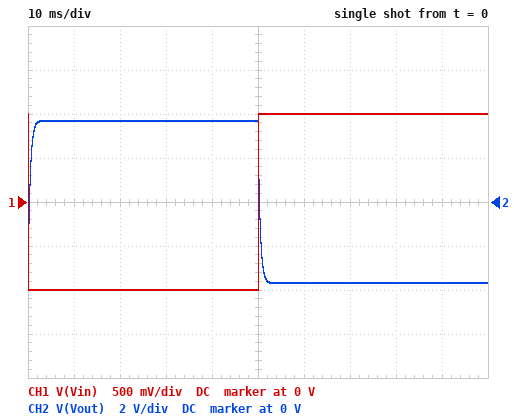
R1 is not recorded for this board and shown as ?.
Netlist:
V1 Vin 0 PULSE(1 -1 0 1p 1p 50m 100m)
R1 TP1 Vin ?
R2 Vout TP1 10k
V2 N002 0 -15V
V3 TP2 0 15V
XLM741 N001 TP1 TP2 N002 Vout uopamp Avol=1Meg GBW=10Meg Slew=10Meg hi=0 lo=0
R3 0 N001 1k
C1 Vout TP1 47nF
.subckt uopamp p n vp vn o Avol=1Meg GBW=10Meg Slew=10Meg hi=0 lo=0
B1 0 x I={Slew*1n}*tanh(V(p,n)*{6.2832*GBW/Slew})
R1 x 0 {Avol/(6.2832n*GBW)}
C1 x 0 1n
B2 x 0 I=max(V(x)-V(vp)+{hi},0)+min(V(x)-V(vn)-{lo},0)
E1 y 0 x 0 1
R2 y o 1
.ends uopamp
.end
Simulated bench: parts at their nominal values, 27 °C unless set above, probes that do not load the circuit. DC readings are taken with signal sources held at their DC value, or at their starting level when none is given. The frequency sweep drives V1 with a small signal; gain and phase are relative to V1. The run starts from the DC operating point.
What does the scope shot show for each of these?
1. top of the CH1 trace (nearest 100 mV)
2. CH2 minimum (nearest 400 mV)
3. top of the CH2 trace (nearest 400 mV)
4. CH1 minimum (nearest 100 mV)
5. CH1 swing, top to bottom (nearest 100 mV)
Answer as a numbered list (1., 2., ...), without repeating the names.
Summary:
1. 1.0 V
2. -3.6 V
3. 3.6 V
4. -1.0 V
5. 2.0 V
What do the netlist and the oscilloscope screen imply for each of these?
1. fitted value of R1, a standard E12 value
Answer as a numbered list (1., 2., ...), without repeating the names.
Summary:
1. 2.7 kΩ
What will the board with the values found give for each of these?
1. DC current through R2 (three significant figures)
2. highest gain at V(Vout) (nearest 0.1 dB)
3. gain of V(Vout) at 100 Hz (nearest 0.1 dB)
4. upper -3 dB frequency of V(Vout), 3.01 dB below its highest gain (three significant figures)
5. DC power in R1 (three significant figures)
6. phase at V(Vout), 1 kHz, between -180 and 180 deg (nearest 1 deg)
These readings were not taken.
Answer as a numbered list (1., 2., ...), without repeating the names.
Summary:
1. 370 µA
2. 11.4 dB
3. 11.0 dB
4. 339 Hz
5. 370 µW
6. 109 deg
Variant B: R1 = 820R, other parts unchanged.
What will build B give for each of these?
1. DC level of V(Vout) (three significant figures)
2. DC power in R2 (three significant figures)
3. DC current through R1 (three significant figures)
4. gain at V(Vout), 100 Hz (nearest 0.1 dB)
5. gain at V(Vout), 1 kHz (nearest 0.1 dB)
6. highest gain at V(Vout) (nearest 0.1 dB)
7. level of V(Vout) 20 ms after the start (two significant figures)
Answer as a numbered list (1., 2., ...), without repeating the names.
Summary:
1. -12.2 V
2. 14.9 mW
3. 1.22 mA
4. 21.4 dB
5. 11.8 dB
6. 21.7 dB
7. 12 V
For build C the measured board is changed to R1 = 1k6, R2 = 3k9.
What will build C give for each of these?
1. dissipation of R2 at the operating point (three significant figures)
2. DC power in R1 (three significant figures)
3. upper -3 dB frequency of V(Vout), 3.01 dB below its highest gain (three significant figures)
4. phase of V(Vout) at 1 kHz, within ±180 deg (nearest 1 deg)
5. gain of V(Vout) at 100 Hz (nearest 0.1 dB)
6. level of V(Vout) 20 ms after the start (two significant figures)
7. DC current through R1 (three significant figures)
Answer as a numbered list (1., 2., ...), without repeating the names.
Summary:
1. 1.52 mW
2. 625 µW
3. 868 Hz
4. 131 deg
5. 7.7 dB
6. 2.4 V
7. 625 µA
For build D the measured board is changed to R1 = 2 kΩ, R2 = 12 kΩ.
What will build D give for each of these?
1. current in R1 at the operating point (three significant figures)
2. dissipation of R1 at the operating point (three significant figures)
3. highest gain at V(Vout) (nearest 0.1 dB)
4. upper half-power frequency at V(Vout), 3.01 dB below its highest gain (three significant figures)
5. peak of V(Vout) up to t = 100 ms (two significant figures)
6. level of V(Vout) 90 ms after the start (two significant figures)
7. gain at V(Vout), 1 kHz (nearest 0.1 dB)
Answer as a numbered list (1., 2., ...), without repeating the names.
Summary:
1. 500 µA
2. 500 µW
3. 15.6 dB
4. 282 Hz
5. 6.0 V
6. -6.0 V
7. 4.2 dB
